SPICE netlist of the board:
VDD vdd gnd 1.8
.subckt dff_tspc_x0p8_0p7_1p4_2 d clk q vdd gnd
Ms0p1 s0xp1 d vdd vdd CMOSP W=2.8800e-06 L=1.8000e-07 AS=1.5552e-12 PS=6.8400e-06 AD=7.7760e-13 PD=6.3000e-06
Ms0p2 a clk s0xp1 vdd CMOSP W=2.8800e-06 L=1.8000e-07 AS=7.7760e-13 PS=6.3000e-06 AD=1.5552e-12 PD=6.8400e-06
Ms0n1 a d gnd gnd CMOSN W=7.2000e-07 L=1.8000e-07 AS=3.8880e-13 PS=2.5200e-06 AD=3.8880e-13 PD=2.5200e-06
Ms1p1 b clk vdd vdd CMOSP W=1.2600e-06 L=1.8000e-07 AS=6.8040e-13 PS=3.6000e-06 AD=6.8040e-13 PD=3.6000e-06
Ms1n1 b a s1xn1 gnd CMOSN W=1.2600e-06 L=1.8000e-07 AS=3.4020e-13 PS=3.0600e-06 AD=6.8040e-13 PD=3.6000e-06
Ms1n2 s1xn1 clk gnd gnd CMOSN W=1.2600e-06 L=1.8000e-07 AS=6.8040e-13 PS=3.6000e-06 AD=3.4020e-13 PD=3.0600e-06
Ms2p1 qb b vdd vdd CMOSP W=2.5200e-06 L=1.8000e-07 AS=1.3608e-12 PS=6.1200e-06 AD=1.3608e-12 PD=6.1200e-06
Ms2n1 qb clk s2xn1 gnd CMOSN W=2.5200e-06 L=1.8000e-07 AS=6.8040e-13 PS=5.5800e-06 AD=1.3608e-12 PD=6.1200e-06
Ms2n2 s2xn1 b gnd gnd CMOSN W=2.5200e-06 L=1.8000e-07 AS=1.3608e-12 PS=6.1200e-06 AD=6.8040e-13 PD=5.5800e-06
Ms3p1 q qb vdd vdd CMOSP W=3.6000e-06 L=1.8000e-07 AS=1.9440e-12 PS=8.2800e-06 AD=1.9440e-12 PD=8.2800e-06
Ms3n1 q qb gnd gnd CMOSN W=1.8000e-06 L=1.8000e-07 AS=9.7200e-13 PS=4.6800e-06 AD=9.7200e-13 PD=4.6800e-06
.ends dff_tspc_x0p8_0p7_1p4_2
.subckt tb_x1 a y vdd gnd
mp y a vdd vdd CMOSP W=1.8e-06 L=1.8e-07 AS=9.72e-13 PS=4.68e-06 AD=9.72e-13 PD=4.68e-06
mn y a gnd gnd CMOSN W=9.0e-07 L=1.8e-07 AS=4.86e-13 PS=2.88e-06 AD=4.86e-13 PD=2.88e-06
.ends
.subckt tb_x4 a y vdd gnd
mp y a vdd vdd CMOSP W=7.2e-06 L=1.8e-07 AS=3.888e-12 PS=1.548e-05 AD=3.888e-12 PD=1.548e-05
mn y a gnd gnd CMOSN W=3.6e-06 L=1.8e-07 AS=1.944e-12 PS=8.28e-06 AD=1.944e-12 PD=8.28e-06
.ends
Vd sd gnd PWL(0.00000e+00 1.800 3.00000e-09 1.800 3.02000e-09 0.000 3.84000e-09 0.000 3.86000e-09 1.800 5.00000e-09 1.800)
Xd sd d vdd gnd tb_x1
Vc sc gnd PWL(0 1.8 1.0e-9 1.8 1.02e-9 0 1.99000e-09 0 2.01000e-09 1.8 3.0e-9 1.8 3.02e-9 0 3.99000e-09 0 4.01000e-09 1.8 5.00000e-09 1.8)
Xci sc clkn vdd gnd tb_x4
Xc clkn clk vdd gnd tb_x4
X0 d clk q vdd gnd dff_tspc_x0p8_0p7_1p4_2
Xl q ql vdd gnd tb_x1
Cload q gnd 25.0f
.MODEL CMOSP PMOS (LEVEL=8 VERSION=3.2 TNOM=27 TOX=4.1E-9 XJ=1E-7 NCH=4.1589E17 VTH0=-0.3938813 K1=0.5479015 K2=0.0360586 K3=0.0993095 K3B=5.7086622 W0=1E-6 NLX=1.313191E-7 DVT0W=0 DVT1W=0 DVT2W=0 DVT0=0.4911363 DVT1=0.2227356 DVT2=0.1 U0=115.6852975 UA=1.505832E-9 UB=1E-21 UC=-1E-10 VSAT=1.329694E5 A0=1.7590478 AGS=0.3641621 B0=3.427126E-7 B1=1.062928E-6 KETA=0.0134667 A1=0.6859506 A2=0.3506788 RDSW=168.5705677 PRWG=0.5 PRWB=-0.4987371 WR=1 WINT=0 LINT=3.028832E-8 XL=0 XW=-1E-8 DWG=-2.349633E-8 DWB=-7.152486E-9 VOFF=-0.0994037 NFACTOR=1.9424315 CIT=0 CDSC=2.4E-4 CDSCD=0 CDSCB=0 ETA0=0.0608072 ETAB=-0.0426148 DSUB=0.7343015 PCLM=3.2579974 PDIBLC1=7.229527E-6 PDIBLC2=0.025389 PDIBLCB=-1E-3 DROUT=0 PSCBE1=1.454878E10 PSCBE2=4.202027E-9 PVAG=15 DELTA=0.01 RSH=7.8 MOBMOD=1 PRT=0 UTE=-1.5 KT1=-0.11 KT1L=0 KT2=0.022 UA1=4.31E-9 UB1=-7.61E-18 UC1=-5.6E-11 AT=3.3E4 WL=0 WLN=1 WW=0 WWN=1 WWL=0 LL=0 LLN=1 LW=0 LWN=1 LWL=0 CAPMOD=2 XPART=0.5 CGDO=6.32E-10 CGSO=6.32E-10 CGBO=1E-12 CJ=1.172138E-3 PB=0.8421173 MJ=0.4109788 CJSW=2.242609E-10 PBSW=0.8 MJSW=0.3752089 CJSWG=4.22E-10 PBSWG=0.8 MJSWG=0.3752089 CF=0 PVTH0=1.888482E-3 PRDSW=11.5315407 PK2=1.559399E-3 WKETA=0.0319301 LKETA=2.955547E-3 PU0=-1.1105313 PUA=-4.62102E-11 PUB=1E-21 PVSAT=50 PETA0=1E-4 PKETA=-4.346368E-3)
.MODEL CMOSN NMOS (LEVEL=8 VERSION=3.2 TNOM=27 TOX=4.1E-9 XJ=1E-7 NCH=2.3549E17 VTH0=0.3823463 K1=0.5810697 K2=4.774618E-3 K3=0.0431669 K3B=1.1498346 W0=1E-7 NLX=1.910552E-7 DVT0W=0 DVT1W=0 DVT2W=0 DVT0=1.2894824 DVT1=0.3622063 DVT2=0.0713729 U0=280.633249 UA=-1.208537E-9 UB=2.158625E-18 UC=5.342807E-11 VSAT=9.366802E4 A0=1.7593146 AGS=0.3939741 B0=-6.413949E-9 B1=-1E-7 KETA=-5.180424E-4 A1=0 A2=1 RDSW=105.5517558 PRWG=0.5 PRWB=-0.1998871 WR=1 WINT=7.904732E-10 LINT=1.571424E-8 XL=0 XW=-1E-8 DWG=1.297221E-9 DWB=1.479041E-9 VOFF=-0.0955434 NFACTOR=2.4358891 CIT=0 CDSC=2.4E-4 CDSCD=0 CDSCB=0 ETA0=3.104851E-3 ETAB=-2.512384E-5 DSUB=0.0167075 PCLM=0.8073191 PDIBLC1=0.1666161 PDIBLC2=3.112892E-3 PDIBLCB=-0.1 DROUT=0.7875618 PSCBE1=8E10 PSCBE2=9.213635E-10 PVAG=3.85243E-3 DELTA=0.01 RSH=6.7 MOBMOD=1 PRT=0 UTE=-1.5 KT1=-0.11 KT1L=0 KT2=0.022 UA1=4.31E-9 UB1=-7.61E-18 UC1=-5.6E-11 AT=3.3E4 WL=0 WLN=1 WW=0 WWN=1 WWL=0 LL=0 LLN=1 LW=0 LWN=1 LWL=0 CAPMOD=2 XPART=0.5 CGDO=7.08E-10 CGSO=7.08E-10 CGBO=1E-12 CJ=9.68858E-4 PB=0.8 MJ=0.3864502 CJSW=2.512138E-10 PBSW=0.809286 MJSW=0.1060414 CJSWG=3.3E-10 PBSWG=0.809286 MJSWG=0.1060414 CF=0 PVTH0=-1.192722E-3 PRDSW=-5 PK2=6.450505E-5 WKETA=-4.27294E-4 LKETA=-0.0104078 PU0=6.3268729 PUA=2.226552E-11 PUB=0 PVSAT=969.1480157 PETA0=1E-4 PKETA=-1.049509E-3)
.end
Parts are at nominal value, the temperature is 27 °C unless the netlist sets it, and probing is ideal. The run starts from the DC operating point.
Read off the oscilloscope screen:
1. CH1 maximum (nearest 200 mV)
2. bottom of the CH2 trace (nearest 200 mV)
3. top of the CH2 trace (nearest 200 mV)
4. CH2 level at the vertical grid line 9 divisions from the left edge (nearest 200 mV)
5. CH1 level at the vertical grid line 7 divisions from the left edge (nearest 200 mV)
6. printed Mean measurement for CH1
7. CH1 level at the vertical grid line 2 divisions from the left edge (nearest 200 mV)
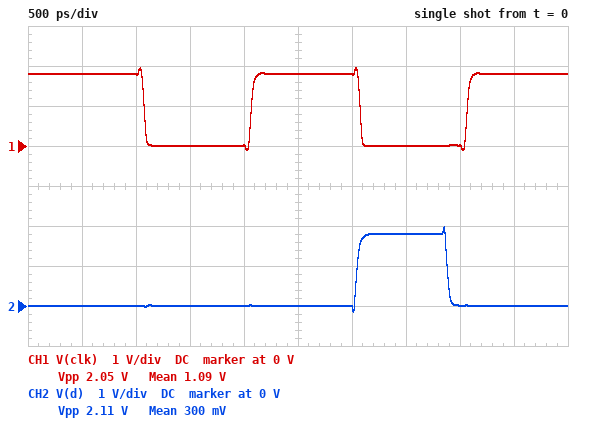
2.0 V
-200 mV
2.0 V
0 V
0 V
1.09 V
1.8 V
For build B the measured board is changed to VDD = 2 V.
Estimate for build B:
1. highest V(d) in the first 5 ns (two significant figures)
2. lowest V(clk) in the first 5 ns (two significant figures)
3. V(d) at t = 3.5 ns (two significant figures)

2.2 V
-97 mV
2.0 V
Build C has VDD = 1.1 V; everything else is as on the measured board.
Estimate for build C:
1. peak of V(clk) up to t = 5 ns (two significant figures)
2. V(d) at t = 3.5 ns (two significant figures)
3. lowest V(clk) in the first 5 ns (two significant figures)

1.2 V
1.1 V
-190 mV
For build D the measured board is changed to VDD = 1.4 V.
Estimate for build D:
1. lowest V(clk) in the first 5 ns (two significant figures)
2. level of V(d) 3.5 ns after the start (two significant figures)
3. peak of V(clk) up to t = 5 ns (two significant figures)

-150 mV
1.4 V
1.5 V
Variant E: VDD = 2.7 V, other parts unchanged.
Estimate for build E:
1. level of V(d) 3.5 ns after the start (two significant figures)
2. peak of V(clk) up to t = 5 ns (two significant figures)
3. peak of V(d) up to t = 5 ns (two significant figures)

2.7 V
2.9 V
2.8 V
